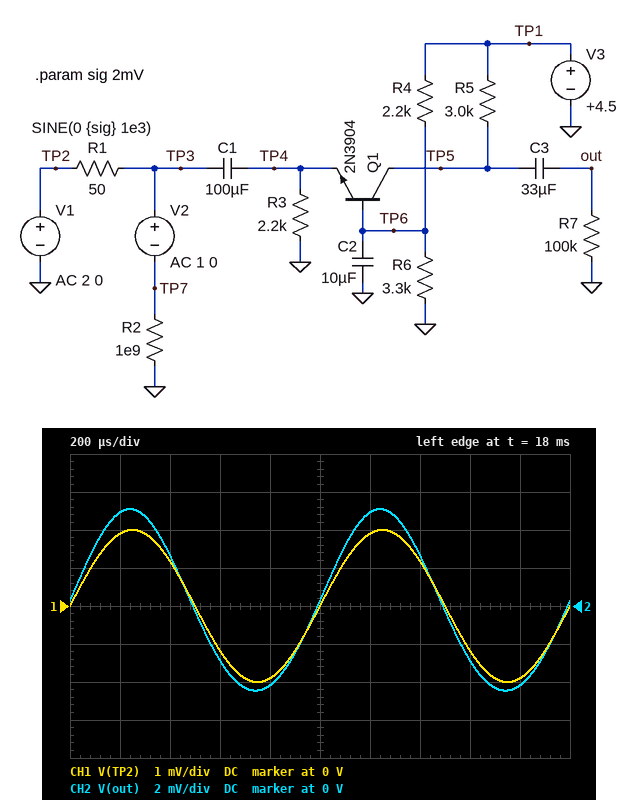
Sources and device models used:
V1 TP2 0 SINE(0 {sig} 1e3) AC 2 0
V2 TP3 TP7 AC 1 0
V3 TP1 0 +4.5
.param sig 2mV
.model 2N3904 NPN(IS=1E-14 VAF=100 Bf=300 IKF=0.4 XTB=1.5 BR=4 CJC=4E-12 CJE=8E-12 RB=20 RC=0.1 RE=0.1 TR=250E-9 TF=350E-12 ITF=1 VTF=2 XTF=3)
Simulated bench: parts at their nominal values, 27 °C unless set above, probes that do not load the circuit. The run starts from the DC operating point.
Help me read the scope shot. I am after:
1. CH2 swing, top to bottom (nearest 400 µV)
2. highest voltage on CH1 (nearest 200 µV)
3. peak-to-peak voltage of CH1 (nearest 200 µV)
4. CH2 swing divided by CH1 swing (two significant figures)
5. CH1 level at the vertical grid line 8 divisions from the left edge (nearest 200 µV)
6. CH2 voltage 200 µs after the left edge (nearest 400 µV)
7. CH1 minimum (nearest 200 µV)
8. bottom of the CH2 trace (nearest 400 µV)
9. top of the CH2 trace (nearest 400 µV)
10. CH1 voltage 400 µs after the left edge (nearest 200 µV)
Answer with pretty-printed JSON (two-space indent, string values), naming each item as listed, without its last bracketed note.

{
  "CH2 swing, top to bottom": "9.6 mV",
  "highest voltage on CH1": "2.0 mV",
  "peak-to-peak voltage of CH1": "4.0 mV",
  "CH2 swing divided by CH1 swing": "2.4",
  "CH1 level at the vertical grid line 8 divisions from the left edge": "-1.2 mV",
  "CH2 voltage 200 µs after the left edge": "4.8 mV",
  "CH1 minimum": "-2.0 mV",
  "bottom of the CH2 trace": "-4.4 mV",
  "top of the CH2 trace": "5.2 mV",
  "CH1 voltage 400 µs after the left edge": "1.2 mV"
}
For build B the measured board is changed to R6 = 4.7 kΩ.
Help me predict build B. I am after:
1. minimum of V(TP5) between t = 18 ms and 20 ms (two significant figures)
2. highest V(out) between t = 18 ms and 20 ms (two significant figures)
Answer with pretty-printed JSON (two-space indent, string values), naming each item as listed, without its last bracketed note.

{
  "minimum of V(TP5) between t = 18 ms and 20 ms": "2.1 V",
  "highest V(out) between t = 18 ms and 20 ms": "2.2 mV"
}
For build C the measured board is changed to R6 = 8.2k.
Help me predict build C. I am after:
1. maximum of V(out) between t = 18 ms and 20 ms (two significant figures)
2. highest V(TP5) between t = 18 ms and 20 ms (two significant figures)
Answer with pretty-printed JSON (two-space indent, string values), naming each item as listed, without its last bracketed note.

{
  "maximum of V(out) between t = 18 ms and 20 ms": "1.6 mV",
  "highest V(TP5) between t = 18 ms and 20 ms": "2.3 V"
}
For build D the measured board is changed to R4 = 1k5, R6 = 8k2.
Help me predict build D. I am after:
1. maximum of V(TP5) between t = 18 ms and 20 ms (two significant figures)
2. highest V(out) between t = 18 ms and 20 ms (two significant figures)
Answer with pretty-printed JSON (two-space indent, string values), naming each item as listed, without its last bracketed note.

{
  "maximum of V(TP5) between t = 18 ms and 20 ms": "2.5 V",
  "highest V(out) between t = 18 ms and 20 ms": "1.3 mV"
}
